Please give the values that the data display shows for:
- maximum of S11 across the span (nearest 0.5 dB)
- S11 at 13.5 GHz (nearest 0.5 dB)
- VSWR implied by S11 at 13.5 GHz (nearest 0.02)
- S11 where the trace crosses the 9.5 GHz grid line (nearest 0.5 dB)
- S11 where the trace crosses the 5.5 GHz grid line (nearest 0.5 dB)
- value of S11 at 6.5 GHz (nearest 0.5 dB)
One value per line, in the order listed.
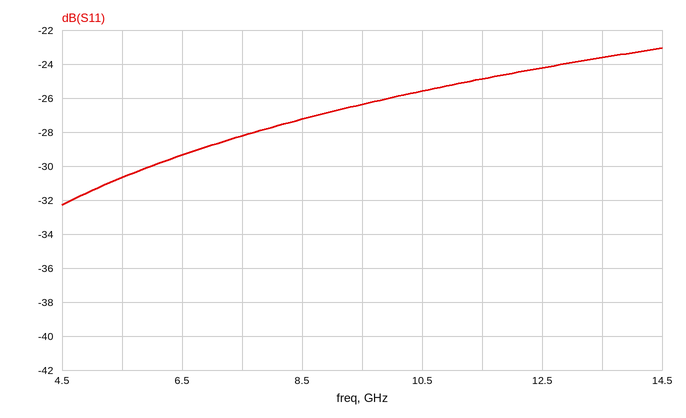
-23.0 dB
-23.5 dB
1.14
-26.5 dB
-30.5 dB
-29.5 dB
